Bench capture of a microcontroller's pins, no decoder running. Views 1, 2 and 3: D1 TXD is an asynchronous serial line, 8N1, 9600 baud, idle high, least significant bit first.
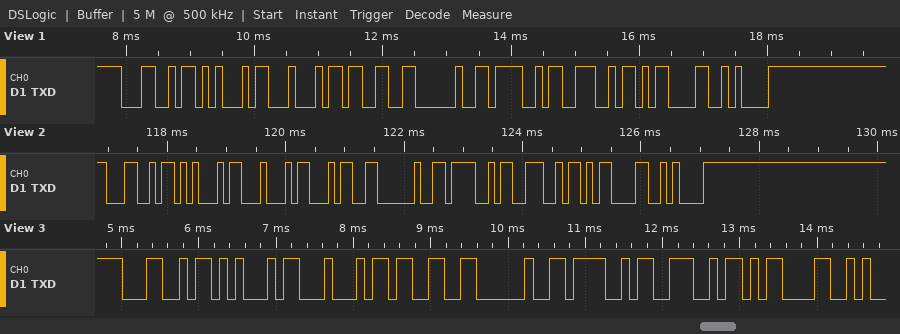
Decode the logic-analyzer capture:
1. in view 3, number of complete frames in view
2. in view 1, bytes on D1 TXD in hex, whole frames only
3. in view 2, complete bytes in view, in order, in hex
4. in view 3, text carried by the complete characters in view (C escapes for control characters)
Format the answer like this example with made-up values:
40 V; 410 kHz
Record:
8; 0x4C 0x45 0x44 0x33 0x20 0x4F 0x4E 0x0D 0x0A; 4C 45 44 34 20 4F 4E 0D 0A; "LED3 ON\r"
